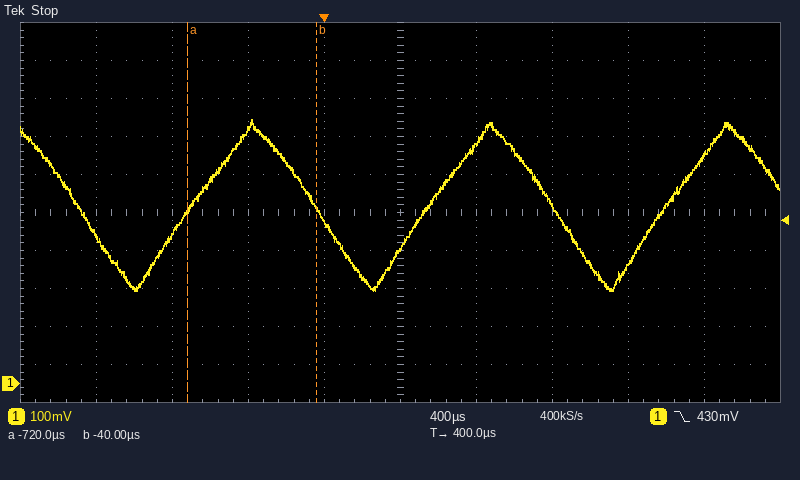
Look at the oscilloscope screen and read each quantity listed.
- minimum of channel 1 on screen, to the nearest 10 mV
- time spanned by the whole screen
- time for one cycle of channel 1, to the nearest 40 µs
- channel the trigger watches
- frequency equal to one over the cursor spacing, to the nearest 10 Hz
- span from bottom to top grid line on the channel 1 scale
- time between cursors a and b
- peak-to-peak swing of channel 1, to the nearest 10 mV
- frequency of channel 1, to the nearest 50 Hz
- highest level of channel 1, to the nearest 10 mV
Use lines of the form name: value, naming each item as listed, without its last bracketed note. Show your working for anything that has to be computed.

minimum of channel 1 on screen, to the nearest 10 mV: 240 mV
time spanned by the whole screen: 4 ms
time for one cycle of channel 1, to the nearest 40 µs: 1.24 ms
channel the trigger watches: channel 1
frequency equal to one over the cursor spacing, to the nearest 10 Hz: 1 / 680 µs ≈ 1.47 kHz
span from bottom to top grid line on the channel 1 scale: 1 V
time between cursors a and b: -40 µs − (-720 µs) = 680 µs
peak-to-peak swing of channel 1, to the nearest 10 mV: 690 mV − (240 mV) = 450 mV
frequency of channel 1, to the nearest 50 Hz: 1 / 1.24 ms ≈ 806 Hz, so 800 Hz to the nearest 50 Hz
highest level of channel 1, to the nearest 10 mV: 690 mV
